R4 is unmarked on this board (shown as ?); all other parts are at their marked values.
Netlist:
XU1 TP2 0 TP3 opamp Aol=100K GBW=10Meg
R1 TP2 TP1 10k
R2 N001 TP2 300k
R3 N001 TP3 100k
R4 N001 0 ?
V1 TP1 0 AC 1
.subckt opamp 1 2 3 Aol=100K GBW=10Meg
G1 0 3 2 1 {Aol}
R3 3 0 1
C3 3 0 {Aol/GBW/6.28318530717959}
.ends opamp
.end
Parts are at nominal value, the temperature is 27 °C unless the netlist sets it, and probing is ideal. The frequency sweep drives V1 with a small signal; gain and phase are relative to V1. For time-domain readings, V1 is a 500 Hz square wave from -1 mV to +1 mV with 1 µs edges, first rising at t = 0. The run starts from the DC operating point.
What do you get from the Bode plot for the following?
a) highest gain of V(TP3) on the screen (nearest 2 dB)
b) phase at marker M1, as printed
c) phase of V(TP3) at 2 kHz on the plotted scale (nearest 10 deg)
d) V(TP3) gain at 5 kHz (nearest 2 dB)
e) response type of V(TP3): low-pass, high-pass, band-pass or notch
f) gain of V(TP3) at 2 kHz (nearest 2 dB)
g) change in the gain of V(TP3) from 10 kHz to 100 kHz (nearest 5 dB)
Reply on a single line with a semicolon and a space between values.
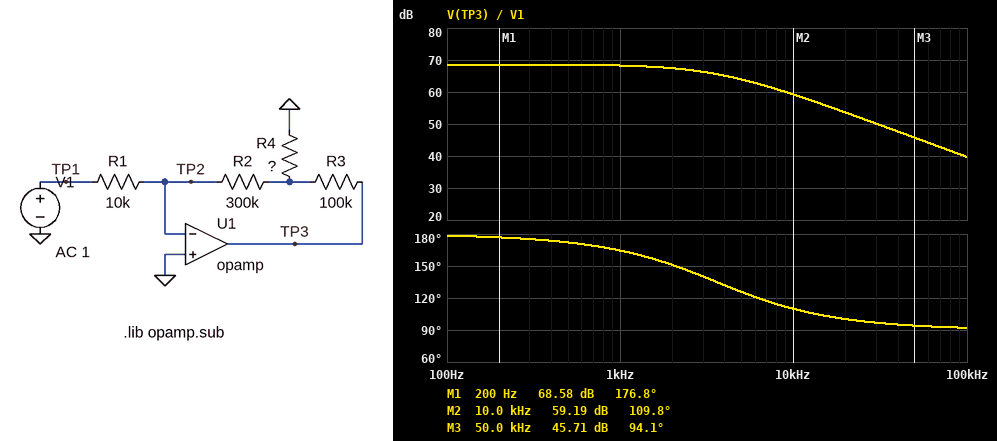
68 dB; 176.8 deg; 150 deg; 64 dB; low-pass; 68 dB; -20 dB
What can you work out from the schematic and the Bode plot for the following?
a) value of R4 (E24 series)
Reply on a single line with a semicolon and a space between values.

1.1 kΩ
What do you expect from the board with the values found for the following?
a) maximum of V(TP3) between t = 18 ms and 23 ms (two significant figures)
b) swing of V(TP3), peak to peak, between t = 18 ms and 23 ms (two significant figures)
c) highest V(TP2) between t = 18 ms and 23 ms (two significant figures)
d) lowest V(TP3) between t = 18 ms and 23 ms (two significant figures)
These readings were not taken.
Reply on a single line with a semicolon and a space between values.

2.7 V; 5.4 V; 1.9 mV; -2.7 V
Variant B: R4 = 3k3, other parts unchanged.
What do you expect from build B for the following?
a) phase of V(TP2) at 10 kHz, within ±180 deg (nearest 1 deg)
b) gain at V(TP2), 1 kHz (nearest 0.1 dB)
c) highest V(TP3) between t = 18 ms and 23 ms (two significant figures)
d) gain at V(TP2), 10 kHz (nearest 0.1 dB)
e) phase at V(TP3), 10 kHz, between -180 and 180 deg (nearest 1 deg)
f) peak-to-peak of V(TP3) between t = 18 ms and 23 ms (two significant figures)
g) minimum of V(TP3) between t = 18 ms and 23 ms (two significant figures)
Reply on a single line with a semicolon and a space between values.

45 deg; -20.5 dB; 940 mV; -3.4 dB; 136 deg; 1.9 V; -940 mV
